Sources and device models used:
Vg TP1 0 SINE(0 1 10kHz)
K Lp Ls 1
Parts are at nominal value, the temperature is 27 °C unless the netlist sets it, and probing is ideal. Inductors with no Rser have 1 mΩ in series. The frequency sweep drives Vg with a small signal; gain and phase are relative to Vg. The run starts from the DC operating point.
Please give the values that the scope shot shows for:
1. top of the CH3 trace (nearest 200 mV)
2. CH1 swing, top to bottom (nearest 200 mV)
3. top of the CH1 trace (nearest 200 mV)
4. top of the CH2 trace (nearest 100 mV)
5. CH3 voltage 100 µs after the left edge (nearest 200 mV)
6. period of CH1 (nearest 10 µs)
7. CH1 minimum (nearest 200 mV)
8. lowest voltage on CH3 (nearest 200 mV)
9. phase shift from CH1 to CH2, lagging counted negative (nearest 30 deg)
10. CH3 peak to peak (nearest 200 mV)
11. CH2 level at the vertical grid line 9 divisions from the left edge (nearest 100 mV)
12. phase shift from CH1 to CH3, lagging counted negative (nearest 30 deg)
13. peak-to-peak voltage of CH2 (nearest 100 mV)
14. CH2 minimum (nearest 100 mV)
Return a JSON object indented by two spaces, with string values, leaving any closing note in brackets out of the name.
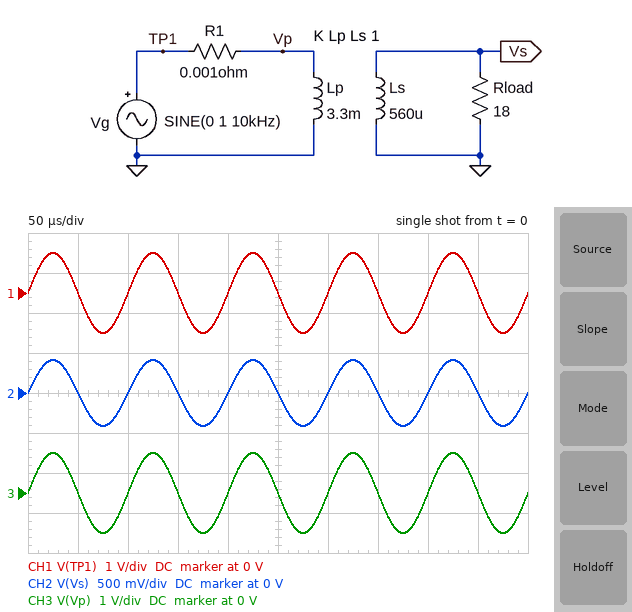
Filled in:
{
  "top of the CH3 trace": "1.0 V",
  "CH1 swing, top to bottom": "2.0 V",
  "top of the CH1 trace": "1.0 V",
  "top of the CH2 trace": "400 mV",
  "CH3 voltage 100 µs after the left edge": "0 V",
  "period of CH1": "100 µs",
  "CH1 minimum": "-1.0 V",
  "lowest voltage on CH3": "-1.0 V",
  "phase shift from CH1 to CH2, lagging counted negative": "0 deg",
  "CH3 peak to peak": "2.0 V",
  "CH2 level at the vertical grid line 9 divisions from the left edge": "0 V",
  "phase shift from CH1 to CH3, lagging counted negative": "0 deg",
  "peak-to-peak voltage of CH2": "800 mV",
  "CH2 minimum": "-400 mV"
}
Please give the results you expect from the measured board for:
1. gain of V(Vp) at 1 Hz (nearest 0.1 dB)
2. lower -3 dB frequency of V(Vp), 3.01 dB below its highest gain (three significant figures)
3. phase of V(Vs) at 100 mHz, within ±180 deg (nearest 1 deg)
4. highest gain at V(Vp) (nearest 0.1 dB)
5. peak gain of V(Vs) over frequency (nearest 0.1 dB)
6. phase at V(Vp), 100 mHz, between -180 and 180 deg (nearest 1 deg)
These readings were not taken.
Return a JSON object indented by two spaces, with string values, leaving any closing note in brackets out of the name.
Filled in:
{
  "gain of V(Vp) at 1 Hz": "0 dB",
  "lower -3 dB frequency of V(Vp), 3.01 dB below its highest gain": "68.2 mHz",
  "phase of V(Vs) at 100 mHz, within ±180 deg": "44 deg",
  "highest gain at V(Vp)": "0 dB",
  "peak gain of V(Vs) over frequency": "-7.7 dB",
  "phase at V(Vp), 100 mHz, between -180 and 180 deg": "18 deg"
}
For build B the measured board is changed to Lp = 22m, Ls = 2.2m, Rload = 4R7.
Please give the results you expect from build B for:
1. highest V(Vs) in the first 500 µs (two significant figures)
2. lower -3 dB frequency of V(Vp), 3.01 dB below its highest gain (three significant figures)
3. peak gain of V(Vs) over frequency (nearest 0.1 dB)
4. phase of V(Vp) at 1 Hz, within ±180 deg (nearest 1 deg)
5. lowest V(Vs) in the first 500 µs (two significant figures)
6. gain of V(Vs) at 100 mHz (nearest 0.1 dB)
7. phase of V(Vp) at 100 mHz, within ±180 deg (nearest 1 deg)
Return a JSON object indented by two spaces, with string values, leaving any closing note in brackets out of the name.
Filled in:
{
  "highest V(Vs) in the first 500 µs": "320 mV",
  "lower -3 dB frequency of V(Vp), 3.01 dB below its highest gain": "10.2 mHz",
  "peak gain of V(Vs) over frequency": "-10.0 dB",
  "phase of V(Vp) at 1 Hz, within ±180 deg": "0 deg",
  "lowest V(Vs) in the first 500 µs": "-320 mV",
  "gain of V(Vs) at 100 mHz": "-10.1 dB",
  "phase of V(Vp) at 100 mHz, within ±180 deg": "4 deg"
}
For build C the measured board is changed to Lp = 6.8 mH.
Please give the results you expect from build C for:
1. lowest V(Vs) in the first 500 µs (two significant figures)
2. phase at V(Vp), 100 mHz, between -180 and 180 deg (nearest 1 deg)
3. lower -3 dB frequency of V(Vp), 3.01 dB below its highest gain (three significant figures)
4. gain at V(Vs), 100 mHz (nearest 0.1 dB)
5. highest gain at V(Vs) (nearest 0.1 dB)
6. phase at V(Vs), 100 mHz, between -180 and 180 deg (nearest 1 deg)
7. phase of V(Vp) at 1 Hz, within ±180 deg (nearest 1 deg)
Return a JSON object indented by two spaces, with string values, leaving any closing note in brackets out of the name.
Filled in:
{
  "lowest V(Vs) in the first 500 µs": "-290 mV",
  "phase at V(Vp), 100 mHz, between -180 and 180 deg": "12 deg",
  "lower -3 dB frequency of V(Vp), 3.01 dB below its highest gain": "33.1 mHz",
  "gain at V(Vs), 100 mHz": "-11.7 dB",
  "highest gain at V(Vs)": "-10.8 dB",
  "phase at V(Vs), 100 mHz, between -180 and 180 deg": "25 deg",
  "phase of V(Vp) at 1 Hz, within ±180 deg": "1 deg"
}
